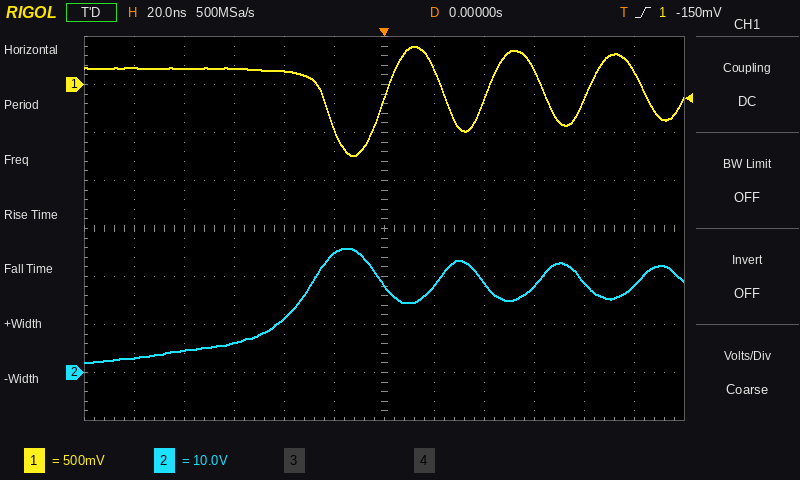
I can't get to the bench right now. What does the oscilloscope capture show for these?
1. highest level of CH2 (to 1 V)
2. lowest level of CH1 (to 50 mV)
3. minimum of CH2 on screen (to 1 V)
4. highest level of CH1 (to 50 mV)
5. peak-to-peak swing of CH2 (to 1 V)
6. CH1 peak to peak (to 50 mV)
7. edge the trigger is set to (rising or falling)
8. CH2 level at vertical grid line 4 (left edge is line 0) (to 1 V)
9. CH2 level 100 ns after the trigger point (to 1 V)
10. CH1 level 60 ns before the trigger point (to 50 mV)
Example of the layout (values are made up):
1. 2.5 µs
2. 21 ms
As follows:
1. 26 V
2. -750 mV
3. 2 V
4. 400 mV
5. 24 V
6. 1.15 V
7. rising
8. 11 V
9. 18 V
10. 150 mV
